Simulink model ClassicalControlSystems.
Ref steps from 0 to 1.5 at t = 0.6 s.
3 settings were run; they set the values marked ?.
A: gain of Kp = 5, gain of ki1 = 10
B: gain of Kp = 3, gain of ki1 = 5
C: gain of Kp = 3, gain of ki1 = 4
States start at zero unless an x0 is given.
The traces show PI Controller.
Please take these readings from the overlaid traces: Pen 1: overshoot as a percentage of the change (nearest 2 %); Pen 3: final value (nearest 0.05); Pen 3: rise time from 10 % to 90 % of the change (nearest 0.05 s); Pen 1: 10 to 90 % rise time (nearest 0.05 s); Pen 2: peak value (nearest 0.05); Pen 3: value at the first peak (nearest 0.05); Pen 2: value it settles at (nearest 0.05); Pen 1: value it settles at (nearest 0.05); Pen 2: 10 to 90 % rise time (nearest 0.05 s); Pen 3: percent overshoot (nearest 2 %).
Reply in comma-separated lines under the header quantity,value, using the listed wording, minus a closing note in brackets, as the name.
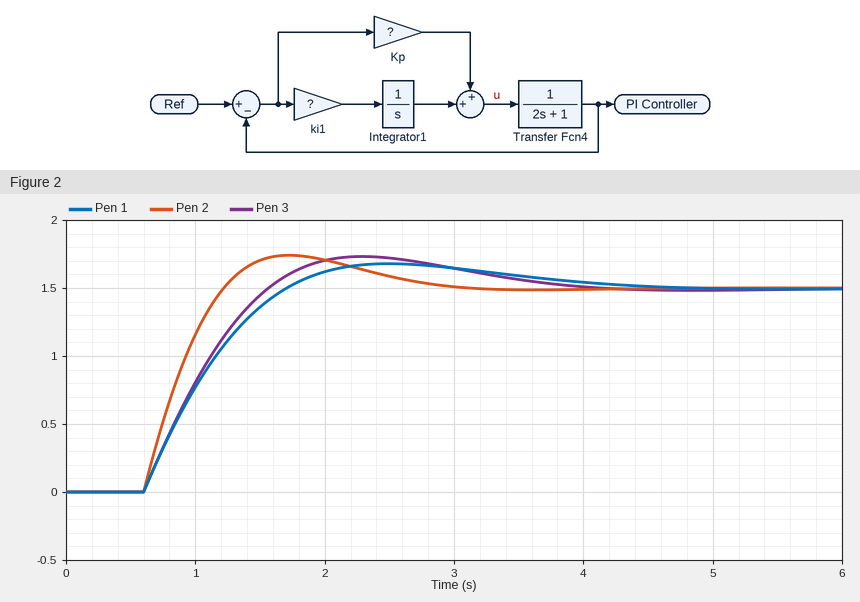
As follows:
quantity,value
Pen 1: overshoot as a percentage of the change,12 %
Pen 3: final value,1.50
Pen 3: rise time from 10 % to 90 % of the change,0.75 s
Pen 1: 10 to 90 % rise time,0.80 s
Pen 2: peak value,1.75
Pen 3: value at the first peak,1.75
Pen 2: value it settles at,1.50
Pen 1: value it settles at,1.50
Pen 2: 10 to 90 % rise time,0.45 s
Pen 3: percent overshoot,16 %
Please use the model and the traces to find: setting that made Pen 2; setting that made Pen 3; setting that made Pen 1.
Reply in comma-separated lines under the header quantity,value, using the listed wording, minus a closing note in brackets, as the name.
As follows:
quantity,value
setting that made Pen 2,A
setting that made Pen 3,B
setting that made Pen 1,C
